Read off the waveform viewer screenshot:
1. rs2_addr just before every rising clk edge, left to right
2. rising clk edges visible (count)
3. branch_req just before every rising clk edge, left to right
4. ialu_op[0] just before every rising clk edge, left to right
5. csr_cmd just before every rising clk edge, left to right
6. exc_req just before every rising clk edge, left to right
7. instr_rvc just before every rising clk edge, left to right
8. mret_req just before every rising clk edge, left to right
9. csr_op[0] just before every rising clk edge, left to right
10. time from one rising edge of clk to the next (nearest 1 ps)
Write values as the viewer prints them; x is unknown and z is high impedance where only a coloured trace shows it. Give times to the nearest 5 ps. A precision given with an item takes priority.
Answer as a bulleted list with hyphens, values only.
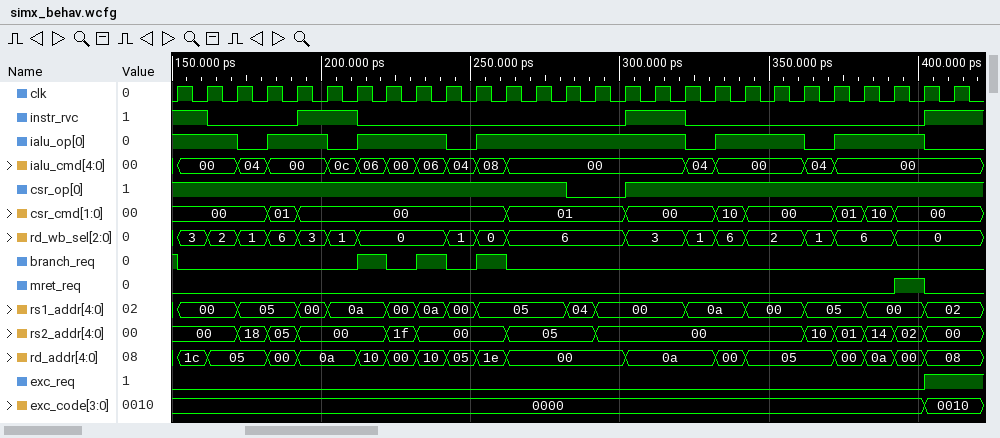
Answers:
- 00, 00, 00, 18, 05, 00, 00, 00, 1f, 00, 00, 00, 05, 05, 05, 00, 00, 00, 00, 00, 00, 00, 10, 01, 14, 02, 00
- 27
- 1 0 0 0 0 0 0 1 0 1 0 1 0 0 0 0 0 0 0 0 0 0 0 0 0 0 0
- 1 1 1 0 1 1 0 1 1 1 0 1 1 1 1 1 1 1 0 1 1 1 0 1 1 1 0
- 00, 00, 00, 00, 01, 00, 00, 00, 00, 00, 00, 00, 01, 01, 01, 01, 00, 00, 00, 10, 00, 00, 00, 01, 10, 00, 00
- 0 0 0 0 0 0 0 0 0 0 0 0 0 0 0 0 0 0 0 0 0 0 0 0 0 0 1
- 1 1 0 0 0 1 1 0 0 0 0 0 0 0 0 0 1 1 0 0 0 0 0 0 0 0 1
- 0 0 0 0 0 0 0 0 0 0 0 0 0 0 0 0 0 0 0 0 0 0 0 0 0 1 0
- 1 1 1 1 1 1 1 1 1 1 1 1 1 1 0 0 1 1 1 1 1 1 1 1 1 1 1
- 10 ps
